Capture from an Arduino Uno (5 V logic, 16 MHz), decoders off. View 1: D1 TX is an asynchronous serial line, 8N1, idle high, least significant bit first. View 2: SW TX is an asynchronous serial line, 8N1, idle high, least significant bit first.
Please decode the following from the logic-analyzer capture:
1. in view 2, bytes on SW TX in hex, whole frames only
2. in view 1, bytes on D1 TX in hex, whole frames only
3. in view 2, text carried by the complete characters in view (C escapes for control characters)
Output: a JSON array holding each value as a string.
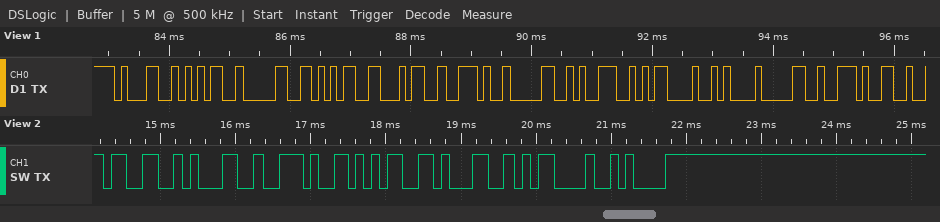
["33 31 2E 35 31 0D 0A", "31 35 30 35 34 2E 30 39 0D 0A 30 2E", "\"31.51\\r\\n\""]
